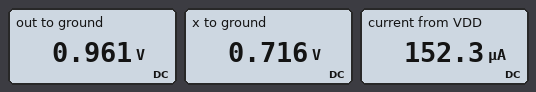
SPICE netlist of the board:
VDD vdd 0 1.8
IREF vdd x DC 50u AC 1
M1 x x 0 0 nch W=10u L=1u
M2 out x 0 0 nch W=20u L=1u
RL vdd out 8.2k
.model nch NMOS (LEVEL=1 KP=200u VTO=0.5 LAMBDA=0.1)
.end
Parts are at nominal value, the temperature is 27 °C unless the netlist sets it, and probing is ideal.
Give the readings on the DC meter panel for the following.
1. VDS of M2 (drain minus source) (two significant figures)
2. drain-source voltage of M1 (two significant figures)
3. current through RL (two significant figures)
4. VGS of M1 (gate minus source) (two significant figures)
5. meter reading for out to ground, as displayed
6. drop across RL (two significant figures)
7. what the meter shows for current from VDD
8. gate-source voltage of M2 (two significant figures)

960 mV
720 mV
100 µA
720 mV
0.961 V
840 mV
152.3 µA
720 mV
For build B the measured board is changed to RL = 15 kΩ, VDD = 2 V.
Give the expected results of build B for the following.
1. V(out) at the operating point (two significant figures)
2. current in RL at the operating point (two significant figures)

530 mV
98 µA
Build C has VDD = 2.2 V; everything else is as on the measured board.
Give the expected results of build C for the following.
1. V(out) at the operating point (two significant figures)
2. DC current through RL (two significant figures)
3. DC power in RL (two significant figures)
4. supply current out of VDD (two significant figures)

1.3 V
110 µA
92 µW
160 µA
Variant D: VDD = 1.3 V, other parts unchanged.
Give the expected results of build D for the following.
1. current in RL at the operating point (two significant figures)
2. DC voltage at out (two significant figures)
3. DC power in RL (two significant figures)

98 µA
500 mV
79 µW
